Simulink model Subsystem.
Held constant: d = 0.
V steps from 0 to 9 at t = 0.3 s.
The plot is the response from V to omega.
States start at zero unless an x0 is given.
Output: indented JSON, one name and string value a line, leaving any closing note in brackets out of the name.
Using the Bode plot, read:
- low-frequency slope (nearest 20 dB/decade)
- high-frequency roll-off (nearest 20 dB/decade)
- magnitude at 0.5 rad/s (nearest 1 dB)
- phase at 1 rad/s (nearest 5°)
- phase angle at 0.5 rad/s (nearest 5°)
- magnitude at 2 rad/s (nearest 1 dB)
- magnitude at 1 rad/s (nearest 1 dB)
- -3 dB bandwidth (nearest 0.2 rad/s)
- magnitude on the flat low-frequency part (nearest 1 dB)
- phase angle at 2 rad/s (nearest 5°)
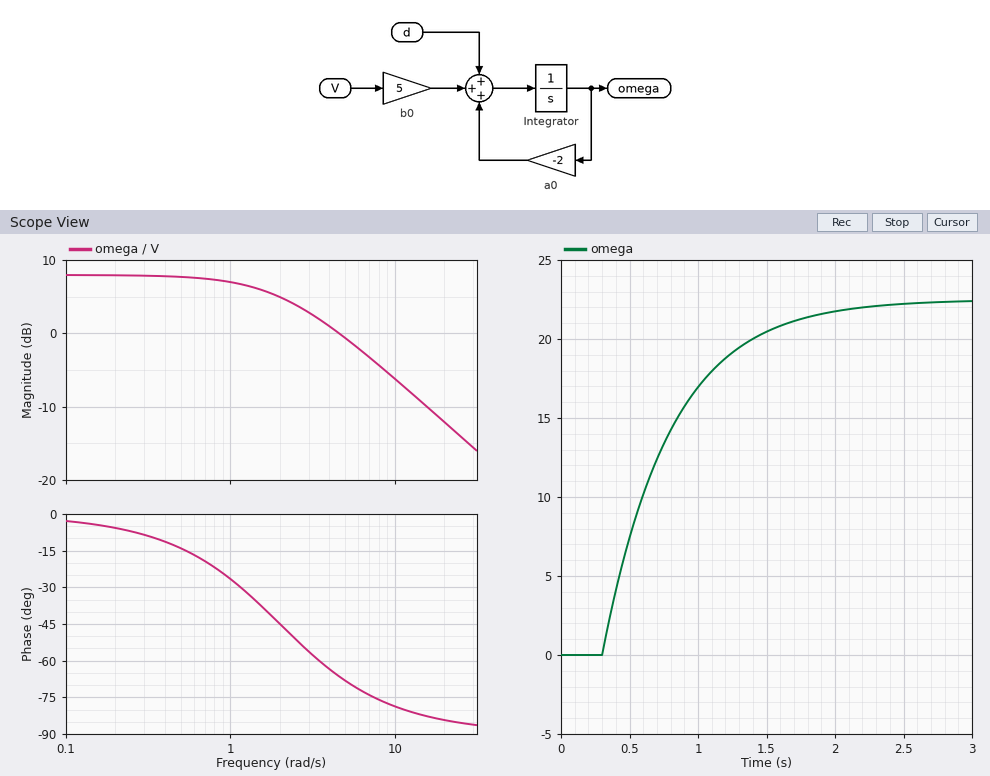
{
  "low-frequency slope": "0 dB/decade",
  "high-frequency roll-off": "-20 dB/decade",
  "magnitude at 0.5 rad/s": "8 dB",
  "phase at 1 rad/s": "-25°",
  "phase angle at 0.5 rad/s": "-15°",
  "magnitude at 2 rad/s": "5 dB",
  "magnitude at 1 rad/s": "7 dB",
  "-3 dB bandwidth": "2.0 rad/s",
  "magnitude on the flat low-frequency part": "8 dB",
  "phase angle at 2 rad/s": "-45°"
}
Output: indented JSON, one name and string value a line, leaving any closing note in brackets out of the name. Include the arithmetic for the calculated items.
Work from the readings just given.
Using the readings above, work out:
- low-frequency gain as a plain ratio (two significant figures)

{
  "low-frequency gain as a plain ratio": "10^(8 / 20) = 2.5"
}
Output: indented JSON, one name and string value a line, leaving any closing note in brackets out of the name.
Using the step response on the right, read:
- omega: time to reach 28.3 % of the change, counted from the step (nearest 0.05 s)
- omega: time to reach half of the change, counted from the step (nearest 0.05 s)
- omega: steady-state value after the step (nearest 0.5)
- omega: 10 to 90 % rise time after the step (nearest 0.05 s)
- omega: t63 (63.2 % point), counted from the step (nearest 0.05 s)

{
  "omega: time to reach 28.3 % of the change, counted from the step": "0.15 s",
  "omega: time to reach half of the change, counted from the step": "0.35 s",
  "omega: steady-state value after the step": "22.5",
  "omega: 10 to 90 % rise time after the step": "1.10 s",
  "omega: t63 (63.2 % point), counted from the step": "0.50 s"
}
